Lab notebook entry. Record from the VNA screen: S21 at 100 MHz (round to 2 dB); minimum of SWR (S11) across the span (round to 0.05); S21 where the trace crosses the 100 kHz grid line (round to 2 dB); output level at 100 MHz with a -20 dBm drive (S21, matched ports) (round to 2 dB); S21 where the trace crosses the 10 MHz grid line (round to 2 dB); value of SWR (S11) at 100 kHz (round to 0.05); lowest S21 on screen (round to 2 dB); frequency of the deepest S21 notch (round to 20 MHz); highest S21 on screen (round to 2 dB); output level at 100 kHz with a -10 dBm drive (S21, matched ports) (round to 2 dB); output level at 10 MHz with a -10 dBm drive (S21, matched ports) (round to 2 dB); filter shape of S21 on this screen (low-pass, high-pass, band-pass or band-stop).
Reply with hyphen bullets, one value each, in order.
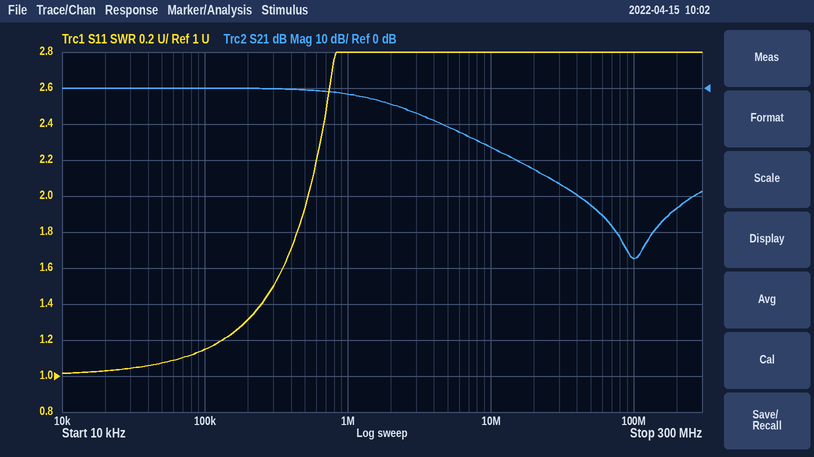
- -48 dB
- 1.00
- 0 dB
- -68 dBm
- -16 dB
- 1.15
- -48 dB
- 100 MHz
- 0 dB
- -10 dBm
- -26 dBm
- low-pass
